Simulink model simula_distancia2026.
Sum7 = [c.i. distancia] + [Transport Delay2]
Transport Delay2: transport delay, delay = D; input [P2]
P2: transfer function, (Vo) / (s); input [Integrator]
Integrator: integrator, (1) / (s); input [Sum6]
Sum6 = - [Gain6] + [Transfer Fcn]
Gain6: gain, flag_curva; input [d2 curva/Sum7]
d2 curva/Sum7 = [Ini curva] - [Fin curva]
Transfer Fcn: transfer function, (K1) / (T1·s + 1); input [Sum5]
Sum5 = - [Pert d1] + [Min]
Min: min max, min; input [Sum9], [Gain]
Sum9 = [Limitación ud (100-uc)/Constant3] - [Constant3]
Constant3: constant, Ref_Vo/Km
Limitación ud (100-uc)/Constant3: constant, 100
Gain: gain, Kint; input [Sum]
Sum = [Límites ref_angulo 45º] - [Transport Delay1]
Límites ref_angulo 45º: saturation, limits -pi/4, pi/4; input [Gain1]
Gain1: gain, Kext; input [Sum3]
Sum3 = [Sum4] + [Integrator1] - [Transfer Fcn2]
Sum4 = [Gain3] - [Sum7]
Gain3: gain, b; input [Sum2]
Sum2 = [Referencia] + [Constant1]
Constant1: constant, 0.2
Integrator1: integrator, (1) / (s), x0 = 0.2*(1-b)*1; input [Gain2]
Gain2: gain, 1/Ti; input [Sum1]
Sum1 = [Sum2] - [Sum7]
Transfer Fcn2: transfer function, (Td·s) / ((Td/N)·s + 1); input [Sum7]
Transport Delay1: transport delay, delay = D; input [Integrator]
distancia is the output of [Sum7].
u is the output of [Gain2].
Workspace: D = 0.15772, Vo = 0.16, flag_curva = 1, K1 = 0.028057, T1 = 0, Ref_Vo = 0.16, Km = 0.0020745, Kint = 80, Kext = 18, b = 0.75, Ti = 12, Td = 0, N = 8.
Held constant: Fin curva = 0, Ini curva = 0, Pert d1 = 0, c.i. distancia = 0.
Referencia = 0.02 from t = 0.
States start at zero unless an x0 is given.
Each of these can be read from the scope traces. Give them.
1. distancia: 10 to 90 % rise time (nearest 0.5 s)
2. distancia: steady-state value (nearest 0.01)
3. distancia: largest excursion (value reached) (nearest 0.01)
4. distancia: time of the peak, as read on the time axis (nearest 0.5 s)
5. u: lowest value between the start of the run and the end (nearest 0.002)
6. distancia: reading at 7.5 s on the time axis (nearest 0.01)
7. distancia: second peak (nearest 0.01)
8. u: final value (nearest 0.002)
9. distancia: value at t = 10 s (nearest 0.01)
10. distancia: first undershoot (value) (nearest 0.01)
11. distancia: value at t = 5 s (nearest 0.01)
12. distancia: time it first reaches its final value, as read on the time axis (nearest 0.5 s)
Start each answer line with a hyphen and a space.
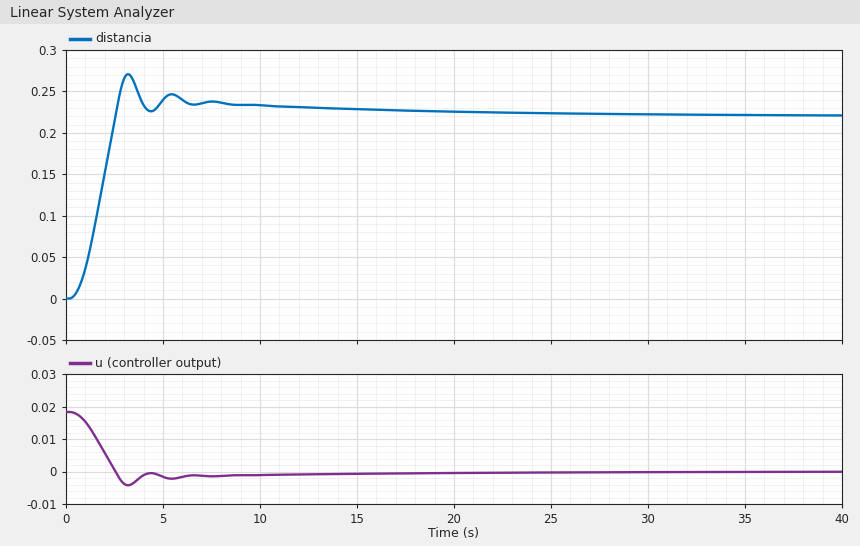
- 1.5 s
- 0.22
- 0.27
- 3.0 s
- -0.004
- 0.24
- 0.25
- 0.000
- 0.23
- 0.23
- 0.24
- 2.5 s
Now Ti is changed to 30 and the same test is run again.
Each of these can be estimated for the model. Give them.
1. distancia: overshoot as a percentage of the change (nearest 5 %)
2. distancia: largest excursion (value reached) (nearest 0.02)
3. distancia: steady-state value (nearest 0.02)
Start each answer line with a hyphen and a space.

- 15 %
- 0.26
- 0.22
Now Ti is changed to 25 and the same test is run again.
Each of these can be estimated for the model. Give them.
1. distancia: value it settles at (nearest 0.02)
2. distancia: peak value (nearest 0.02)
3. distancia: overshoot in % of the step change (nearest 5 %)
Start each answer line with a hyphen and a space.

- 0.22
- 0.26
- 15 %
